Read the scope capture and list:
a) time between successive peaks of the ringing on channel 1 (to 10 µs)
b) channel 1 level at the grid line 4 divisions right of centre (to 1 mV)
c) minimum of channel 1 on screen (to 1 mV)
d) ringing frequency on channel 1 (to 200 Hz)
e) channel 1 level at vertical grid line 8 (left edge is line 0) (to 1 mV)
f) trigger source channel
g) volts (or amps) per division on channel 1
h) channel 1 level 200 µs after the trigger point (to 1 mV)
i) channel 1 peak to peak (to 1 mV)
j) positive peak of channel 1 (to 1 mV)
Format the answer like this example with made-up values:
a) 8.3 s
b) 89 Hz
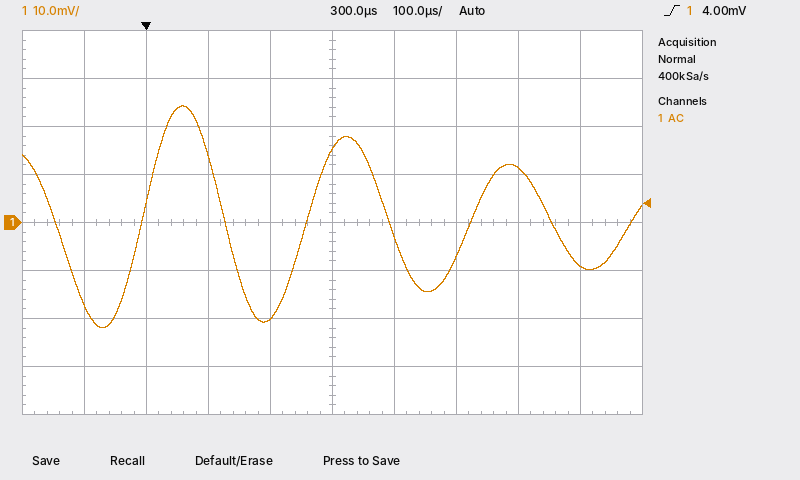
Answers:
a) 260 µs
b) -9 mV
c) -22 mV
d) 3.8 kHz
e) 11 mV
f) channel 1
g) 10 mV
h) -20 mV
i) 46 mV
j) 24 mV
